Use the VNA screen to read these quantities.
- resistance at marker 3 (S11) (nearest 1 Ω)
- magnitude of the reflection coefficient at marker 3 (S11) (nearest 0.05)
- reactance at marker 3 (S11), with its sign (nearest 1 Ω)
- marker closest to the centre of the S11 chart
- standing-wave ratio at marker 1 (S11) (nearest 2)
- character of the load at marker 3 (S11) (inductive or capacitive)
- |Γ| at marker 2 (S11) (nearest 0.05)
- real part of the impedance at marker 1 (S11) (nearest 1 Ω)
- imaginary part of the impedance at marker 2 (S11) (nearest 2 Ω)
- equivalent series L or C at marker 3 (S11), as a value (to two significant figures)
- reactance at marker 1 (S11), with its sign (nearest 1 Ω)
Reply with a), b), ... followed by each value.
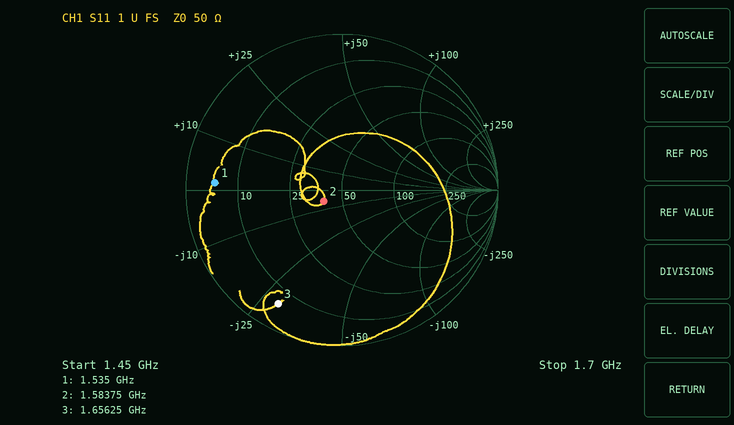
a) 6 Ω
b) 0.85
c) -29 Ω
d) marker 2
e) 10
f) capacitive
g) 0.15
h) 5 Ω
i) -6 Ω
j) 3.3 pF
k) +1 Ω
